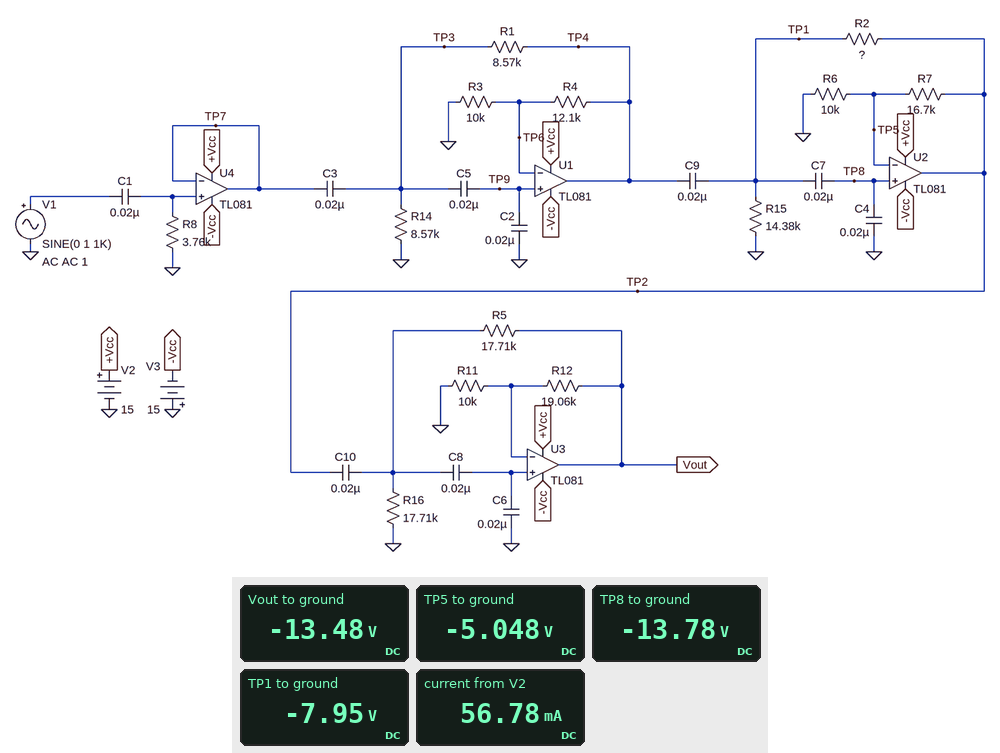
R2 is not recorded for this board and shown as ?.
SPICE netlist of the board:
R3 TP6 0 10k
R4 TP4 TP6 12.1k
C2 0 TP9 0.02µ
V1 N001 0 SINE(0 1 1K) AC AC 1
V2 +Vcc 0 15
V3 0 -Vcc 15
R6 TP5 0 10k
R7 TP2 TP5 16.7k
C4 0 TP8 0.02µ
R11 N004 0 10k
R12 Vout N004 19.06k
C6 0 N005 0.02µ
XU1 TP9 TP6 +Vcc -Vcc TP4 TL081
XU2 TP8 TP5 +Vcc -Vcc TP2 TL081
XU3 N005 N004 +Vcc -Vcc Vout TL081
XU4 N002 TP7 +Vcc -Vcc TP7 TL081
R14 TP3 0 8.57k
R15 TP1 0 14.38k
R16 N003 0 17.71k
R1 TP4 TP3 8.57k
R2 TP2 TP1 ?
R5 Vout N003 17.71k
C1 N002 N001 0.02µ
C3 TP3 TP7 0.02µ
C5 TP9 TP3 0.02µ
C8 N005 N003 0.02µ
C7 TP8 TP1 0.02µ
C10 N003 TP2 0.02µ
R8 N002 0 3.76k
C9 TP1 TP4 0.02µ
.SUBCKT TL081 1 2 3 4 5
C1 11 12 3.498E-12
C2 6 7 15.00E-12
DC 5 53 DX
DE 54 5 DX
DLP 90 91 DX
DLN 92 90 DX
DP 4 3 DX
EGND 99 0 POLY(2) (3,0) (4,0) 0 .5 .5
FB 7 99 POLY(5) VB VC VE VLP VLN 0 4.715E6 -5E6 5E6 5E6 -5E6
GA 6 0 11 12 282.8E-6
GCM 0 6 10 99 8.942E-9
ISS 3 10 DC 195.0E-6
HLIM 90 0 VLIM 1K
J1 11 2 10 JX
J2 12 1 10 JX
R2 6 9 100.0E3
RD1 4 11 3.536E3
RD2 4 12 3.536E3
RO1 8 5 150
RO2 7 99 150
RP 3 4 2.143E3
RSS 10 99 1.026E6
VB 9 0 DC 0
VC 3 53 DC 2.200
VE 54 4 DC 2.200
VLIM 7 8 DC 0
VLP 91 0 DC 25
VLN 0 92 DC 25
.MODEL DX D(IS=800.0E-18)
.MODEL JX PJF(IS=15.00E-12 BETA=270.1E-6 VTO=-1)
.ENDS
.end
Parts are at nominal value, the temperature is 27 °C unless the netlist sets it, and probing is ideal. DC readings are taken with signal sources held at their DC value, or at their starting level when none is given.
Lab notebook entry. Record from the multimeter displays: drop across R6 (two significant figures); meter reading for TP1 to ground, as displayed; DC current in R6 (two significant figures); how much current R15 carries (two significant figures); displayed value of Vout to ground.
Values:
5.0 V
-7.95 V
500 µA
550 µA
-13.48 V
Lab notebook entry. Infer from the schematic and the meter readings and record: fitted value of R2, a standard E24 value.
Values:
10 kΩ
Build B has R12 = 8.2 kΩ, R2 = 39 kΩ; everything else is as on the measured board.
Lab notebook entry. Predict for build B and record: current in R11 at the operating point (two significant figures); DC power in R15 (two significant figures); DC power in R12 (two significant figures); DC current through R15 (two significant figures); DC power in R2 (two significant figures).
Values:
740 µA
920 µW
4.5 mW
250 µA
2.5 mW
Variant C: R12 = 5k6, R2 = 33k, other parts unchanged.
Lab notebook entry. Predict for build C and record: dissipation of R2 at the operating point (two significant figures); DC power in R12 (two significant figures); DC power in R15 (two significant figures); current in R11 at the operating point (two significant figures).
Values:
2.7 mW
4.2 mW
1.2 mW
860 µA
